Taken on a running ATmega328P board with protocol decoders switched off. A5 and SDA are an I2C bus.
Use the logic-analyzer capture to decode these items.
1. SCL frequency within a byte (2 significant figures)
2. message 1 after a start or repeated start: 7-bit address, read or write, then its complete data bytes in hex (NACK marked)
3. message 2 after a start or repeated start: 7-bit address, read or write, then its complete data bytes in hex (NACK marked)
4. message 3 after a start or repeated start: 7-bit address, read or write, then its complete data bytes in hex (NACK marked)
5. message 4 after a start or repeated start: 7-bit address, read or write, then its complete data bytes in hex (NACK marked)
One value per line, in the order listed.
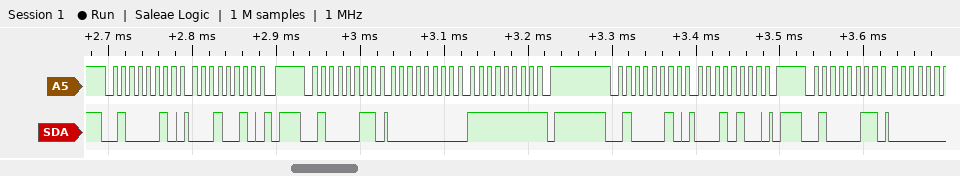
100 kHz
0x21 write: 12
0x21 read: 00 FF NACK
0x21 write: 14
0x21 read
